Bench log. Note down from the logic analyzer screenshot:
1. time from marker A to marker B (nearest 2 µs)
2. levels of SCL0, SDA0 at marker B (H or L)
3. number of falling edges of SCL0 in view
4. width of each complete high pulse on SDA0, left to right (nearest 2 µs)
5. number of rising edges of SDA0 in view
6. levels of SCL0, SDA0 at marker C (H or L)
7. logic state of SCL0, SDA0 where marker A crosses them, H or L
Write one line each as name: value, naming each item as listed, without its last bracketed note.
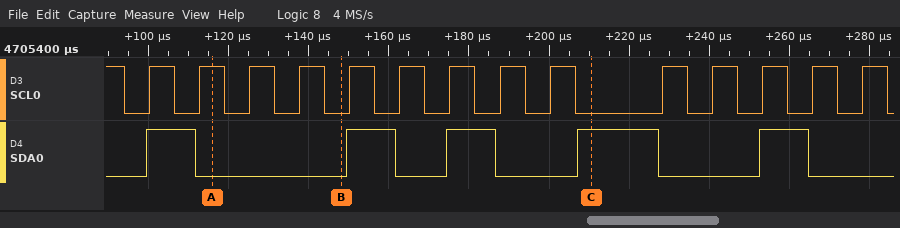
time from marker A to marker B: 32 µs
levels of SCL0, SDA0 at marker B: SCL0=L, SDA0=L
number of falling edges of SCL0 in view: 15
width of each complete high pulse on SDA0, left to right: 12 µs, 12 µs, 12 µs, 20 µs, 12 µs
number of rising edges of SDA0 in view: 5
levels of SCL0, SDA0 at marker C: SCL0=L, SDA0=H
logic state of SCL0, SDA0 where marker A crosses them, H or L: SCL0=H, SDA0=L
